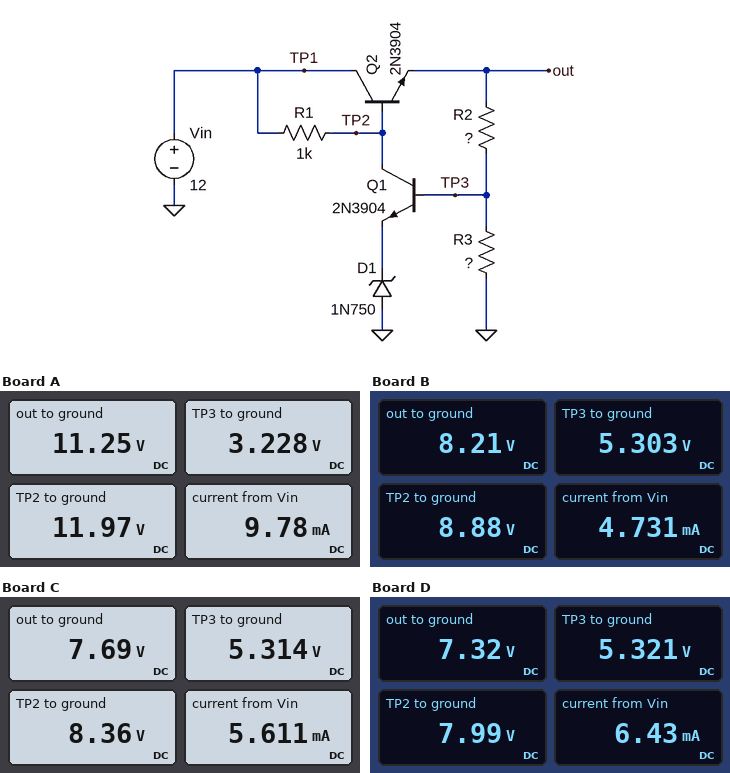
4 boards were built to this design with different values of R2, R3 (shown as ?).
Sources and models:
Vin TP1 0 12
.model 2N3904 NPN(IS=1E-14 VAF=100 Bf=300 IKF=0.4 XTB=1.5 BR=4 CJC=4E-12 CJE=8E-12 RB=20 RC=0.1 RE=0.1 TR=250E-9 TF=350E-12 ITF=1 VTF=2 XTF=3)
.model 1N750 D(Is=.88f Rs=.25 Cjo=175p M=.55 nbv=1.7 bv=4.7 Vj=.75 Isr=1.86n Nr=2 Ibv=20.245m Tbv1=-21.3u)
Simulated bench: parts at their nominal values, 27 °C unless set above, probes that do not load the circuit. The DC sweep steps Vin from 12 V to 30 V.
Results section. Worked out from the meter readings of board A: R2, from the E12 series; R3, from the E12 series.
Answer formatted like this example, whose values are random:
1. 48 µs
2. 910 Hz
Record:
1. 820 Ω
2. 330 Ω
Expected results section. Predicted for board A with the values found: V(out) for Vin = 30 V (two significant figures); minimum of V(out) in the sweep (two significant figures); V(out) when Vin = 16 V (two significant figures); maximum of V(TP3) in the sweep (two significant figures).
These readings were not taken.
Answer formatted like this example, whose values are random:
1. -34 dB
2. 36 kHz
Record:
1. 19 V
2. 11 V
3. 15 V
4. 5.4 V
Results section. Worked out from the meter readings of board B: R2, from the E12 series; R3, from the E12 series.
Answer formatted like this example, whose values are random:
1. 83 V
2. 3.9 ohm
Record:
1. 1.8 kΩ
2. 3.3 kΩ
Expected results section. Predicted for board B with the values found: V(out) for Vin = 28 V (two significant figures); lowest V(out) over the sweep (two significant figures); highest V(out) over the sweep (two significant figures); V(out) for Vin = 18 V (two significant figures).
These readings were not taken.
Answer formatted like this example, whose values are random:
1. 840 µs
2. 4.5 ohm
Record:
1. 8.5 V
2. 8.2 V
3. 8.5 V
4. 8.4 V
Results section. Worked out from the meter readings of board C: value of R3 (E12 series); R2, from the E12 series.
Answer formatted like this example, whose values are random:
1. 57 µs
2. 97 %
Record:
1. 2.7 kΩ
2. 1.2 kΩ
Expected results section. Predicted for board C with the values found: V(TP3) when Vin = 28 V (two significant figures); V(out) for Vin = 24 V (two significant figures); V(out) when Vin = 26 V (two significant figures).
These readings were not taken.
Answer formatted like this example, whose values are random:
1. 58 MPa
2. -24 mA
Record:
1. 5.4 V
2. 7.9 V
3. 7.9 V
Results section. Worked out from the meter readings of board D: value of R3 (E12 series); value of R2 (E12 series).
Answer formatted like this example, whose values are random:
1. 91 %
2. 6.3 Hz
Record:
1. 2.2 kΩ
2. 820 Ω
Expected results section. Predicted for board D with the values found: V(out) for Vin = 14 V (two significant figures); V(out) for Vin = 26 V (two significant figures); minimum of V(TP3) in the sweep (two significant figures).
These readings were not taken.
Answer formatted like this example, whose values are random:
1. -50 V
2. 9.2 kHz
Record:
1. 7.4 V
2. 7.5 V
3. 5.3 V
